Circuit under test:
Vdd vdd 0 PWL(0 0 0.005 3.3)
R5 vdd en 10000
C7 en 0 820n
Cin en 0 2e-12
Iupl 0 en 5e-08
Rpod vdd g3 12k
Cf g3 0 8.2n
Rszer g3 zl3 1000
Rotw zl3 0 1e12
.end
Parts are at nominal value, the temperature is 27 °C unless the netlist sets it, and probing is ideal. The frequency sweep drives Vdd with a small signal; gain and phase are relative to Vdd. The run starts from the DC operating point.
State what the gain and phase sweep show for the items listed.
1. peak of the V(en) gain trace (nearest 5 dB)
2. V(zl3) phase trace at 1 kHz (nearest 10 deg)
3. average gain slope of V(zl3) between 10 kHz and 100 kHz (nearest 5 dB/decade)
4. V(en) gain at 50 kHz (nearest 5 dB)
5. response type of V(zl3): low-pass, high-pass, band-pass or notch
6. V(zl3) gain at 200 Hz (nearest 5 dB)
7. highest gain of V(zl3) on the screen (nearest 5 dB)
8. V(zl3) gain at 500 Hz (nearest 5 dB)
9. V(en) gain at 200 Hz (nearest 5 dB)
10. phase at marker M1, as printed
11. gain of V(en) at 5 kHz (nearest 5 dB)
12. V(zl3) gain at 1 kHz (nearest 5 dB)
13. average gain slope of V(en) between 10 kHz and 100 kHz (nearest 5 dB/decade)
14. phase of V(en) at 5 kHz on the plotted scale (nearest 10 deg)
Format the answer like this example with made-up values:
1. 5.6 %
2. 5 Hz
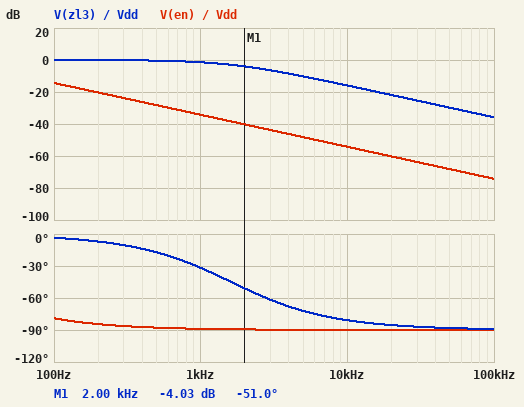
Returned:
1. -15 dB
2. -30 deg
3. -20 dB/decade
4. -70 dB
5. low-pass
6. 0 dB
7. 0 dB
8. 0 dB
9. -20 dB
10. -51.0 deg
11. -50 dB
12. 0 dB
13. -20 dB/decade
14. -90 deg
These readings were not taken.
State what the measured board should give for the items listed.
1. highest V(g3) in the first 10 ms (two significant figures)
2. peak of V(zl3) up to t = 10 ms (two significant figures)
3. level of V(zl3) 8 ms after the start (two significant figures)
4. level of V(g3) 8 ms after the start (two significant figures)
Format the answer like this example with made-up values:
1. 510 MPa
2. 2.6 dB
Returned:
1. 3.3 V
2. 3.3 V
3. 3.3 V
4. 3.3 V
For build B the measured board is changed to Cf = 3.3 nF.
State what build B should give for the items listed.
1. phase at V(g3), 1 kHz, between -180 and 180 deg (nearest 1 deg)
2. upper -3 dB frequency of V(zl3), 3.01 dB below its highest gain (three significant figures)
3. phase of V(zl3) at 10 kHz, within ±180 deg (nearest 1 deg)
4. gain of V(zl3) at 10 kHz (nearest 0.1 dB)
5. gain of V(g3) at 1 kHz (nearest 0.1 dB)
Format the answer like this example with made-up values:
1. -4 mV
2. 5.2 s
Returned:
1. -14 deg
2. 4.02 kHz
3. -68 deg
4. -8.6 dB
5. -0.3 dB
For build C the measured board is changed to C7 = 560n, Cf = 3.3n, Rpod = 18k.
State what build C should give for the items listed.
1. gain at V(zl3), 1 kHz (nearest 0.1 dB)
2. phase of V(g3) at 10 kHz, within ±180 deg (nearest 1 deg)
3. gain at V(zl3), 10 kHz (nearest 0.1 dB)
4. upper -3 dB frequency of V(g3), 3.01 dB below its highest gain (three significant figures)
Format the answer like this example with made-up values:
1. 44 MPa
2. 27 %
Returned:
1. -0.6 dB
2. -75 deg
3. -11.7 dB
4. 2.68 kHz
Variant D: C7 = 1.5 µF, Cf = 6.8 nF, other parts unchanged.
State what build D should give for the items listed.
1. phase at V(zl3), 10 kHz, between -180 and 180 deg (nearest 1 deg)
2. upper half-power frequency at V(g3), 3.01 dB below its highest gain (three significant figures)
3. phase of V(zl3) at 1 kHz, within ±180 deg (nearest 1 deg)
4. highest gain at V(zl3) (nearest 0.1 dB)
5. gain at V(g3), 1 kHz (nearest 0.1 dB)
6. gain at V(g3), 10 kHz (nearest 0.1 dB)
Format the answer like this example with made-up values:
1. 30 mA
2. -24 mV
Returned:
1. -79 deg
2. 1.95 kHz
3. -27 deg
4. 0 dB
5. -1.0 dB
6. -14.4 dB
